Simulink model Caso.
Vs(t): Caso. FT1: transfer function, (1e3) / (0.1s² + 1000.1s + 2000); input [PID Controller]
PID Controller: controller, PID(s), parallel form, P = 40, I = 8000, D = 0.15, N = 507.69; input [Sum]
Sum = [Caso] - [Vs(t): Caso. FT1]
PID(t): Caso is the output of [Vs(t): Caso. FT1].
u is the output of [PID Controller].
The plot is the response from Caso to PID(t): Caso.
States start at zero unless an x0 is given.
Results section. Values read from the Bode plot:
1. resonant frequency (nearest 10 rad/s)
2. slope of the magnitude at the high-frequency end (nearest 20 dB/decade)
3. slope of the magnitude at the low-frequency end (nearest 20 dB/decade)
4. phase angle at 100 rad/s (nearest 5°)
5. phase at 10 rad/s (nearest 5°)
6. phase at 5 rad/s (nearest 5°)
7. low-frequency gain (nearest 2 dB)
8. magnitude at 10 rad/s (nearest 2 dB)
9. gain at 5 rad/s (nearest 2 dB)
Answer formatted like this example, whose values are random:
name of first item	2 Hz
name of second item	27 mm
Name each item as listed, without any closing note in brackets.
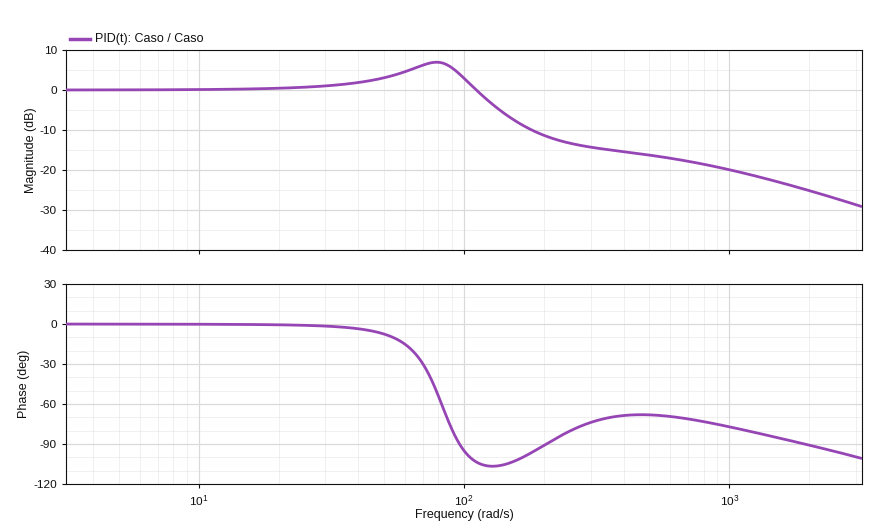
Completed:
resonant frequency	80 rad/s
slope of the magnitude at the high-frequency end	-20 dB/decade
slope of the magnitude at the low-frequency end	0 dB/decade
phase angle at 100 rad/s	-95°
phase at 10 rad/s	0°
phase at 5 rad/s	0°
low-frequency gain	0 dB
magnitude at 10 rad/s	0 dB
gain at 5 rad/s	0 dB
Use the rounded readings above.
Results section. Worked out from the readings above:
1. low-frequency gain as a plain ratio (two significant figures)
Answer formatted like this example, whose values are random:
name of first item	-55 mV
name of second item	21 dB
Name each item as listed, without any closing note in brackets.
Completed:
low-frequency gain as a plain ratio	1.0
